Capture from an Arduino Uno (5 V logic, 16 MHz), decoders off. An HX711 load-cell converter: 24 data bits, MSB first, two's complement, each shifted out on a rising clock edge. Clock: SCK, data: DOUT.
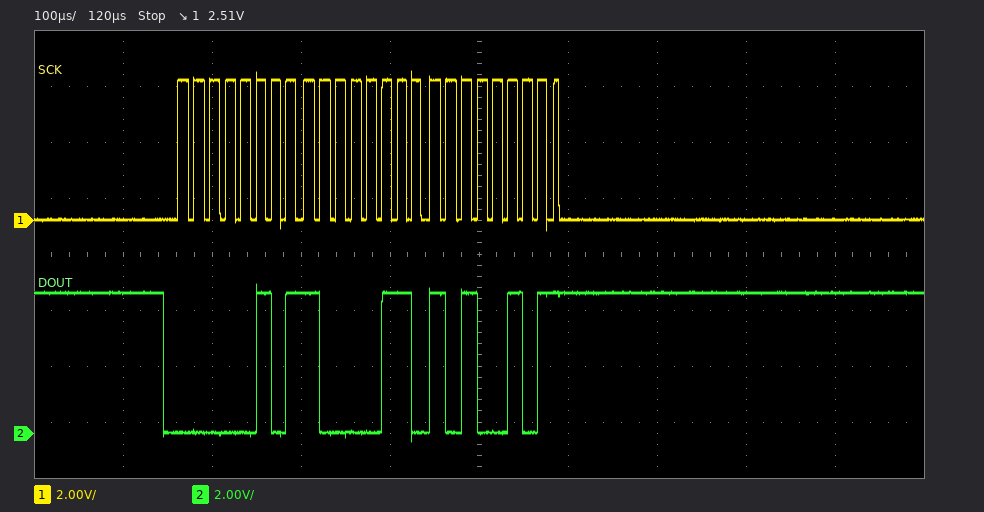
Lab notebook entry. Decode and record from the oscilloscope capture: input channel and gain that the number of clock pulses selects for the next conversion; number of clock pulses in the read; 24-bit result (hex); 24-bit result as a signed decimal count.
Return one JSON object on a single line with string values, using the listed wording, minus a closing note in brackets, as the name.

{"input channel and gain that the number of clock pulses selects for the next conversion": "channel A, gain 128", "number of clock pulses in the read": "25", "24-bit result": "0x0586A5", "24-bit result as a signed decimal count": "362149"}
